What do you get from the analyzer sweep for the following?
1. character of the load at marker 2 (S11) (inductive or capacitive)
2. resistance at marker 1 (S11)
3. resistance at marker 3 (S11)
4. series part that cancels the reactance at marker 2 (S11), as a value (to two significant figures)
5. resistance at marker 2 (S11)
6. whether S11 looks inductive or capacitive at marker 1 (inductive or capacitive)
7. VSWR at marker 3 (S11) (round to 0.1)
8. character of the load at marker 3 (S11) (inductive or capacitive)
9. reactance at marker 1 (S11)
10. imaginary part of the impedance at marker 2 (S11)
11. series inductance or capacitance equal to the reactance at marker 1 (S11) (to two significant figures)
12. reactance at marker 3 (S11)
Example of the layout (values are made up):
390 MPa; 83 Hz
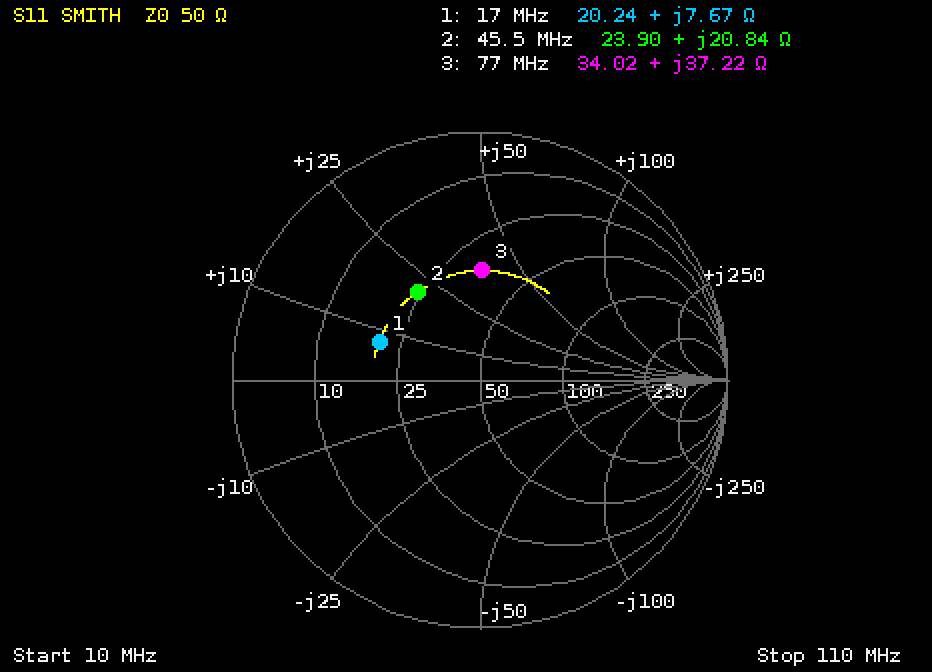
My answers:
inductive; 20.24 Ω; 34.02 Ω; 170 pF; 23.90 Ω; inductive; 2.6; inductive; +7.67 Ω; +20.84 Ω; 72 nH; +37.22 Ω
